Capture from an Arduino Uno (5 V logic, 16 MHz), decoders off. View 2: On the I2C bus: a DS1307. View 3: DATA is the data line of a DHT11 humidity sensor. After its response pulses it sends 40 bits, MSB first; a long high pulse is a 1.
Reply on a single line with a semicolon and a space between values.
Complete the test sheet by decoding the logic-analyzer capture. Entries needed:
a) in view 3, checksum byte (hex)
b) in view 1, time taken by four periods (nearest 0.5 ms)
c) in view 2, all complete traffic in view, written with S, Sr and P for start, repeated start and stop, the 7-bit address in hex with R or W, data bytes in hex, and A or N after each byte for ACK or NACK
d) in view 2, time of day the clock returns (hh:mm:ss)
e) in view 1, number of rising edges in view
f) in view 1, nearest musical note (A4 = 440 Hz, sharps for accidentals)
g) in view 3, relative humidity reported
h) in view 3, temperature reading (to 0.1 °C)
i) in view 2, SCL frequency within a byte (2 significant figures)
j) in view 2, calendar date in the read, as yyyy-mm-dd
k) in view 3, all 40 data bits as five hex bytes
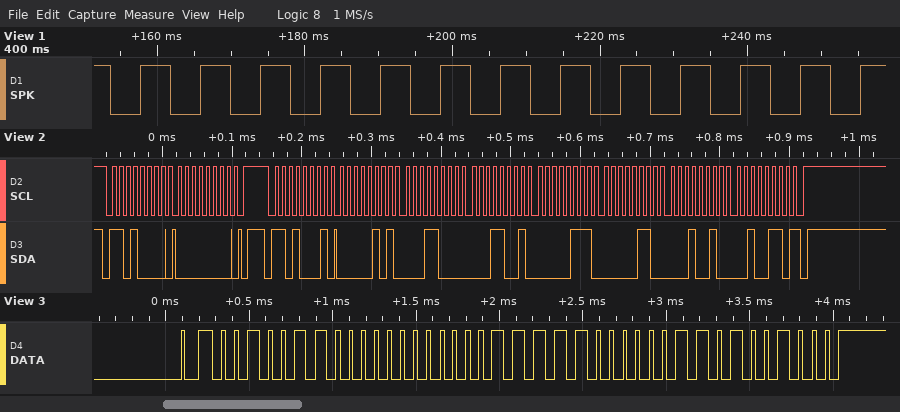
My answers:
0x48; 32.5 ms; S 68W A 00 A P S 68R A 05 A 18 A 19 A 07 A 06 A 12 A 26 N P; 19:18:05; 13; B2; 38 %; 31.3 °C; 100 kHz; 2026-12-06; 26 00 1F 03 48
